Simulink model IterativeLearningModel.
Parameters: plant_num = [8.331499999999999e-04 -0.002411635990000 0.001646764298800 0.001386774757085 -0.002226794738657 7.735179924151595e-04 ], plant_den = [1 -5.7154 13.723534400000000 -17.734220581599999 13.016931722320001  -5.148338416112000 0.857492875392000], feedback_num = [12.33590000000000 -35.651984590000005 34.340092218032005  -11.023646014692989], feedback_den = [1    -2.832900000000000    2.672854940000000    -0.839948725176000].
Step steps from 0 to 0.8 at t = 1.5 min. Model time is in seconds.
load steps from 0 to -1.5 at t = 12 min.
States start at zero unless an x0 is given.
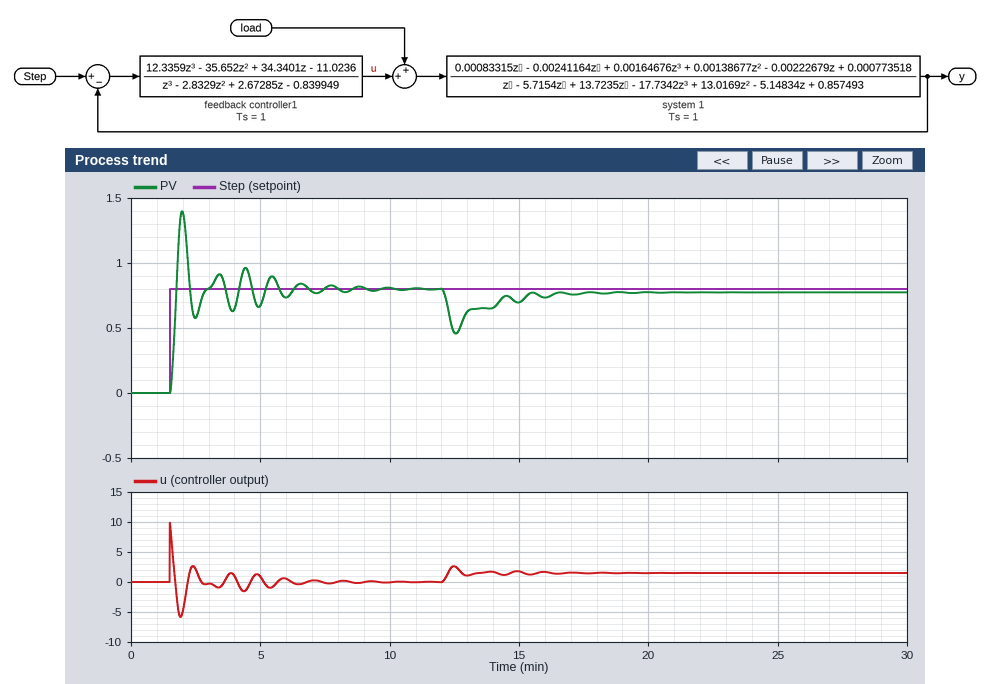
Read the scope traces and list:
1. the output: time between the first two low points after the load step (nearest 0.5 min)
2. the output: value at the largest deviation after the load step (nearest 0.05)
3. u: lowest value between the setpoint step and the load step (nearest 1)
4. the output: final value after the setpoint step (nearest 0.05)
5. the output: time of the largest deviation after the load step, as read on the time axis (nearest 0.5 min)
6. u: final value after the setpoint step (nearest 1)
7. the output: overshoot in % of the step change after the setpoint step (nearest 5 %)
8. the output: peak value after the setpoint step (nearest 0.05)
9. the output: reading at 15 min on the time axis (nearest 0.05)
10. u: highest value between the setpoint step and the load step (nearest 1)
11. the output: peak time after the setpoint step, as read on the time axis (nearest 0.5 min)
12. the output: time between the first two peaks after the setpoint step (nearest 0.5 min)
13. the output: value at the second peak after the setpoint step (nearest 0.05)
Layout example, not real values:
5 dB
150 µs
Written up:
2.5 min
0.45
-6
0.80
12.5 min
0
75 %
1.40
0.70
10
2.0 min
1.5 min
0.90
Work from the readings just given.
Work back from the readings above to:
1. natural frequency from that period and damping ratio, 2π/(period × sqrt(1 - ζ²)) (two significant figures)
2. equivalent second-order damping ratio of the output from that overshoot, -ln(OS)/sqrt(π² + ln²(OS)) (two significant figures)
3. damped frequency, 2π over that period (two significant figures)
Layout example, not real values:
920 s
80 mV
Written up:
4.2 rad/min
0.091
4.2 rad/min
